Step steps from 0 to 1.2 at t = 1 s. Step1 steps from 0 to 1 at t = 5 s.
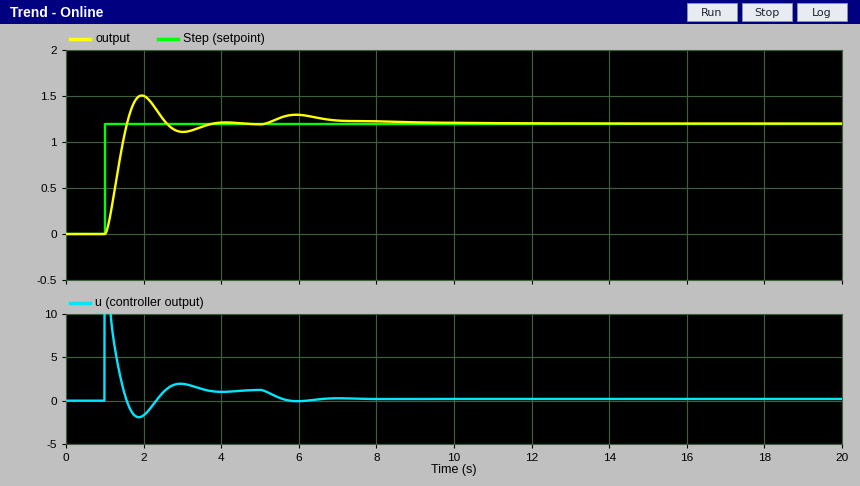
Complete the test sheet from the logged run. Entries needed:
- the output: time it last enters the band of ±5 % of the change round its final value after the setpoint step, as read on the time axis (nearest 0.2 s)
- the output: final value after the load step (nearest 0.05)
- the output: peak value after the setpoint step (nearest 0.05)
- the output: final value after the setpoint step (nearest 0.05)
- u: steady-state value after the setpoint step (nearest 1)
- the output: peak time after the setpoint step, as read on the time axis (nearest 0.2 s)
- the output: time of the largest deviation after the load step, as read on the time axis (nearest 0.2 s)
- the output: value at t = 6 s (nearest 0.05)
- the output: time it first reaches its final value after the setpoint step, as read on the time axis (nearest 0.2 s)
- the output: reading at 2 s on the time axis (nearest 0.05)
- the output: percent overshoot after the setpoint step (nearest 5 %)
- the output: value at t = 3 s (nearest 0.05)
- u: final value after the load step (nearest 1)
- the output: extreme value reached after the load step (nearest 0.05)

3.4 s
1.20
1.50
1.20
1
2.0 s
6.0 s
1.30
1.6 s
1.50
25 %
1.10
0
1.30
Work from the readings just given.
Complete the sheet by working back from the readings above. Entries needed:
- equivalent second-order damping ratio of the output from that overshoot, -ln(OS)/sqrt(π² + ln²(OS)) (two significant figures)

0.40
